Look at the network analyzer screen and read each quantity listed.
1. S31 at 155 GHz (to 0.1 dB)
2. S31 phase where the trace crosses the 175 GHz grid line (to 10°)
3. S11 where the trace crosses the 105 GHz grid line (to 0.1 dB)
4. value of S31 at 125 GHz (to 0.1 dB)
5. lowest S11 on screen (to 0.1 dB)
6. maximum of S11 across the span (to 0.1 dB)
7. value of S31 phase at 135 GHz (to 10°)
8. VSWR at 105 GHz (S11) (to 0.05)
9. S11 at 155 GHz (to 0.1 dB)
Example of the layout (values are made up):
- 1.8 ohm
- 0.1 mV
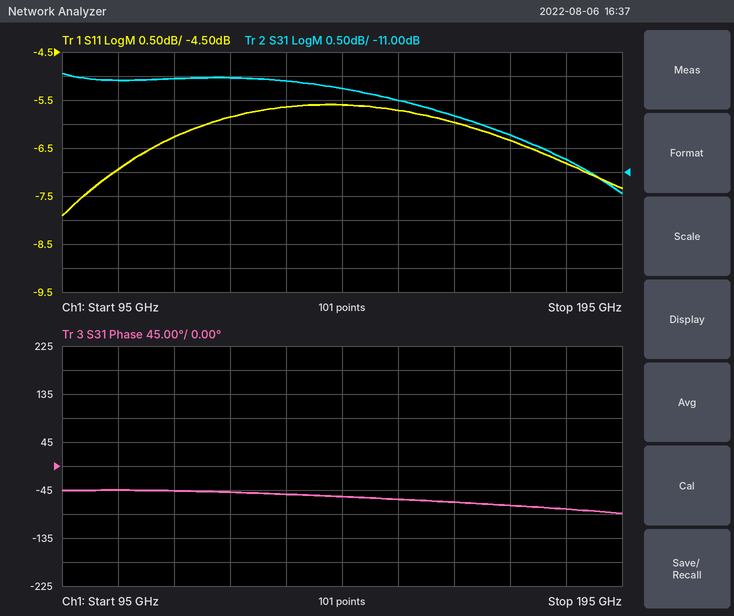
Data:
- -9.5 dB
- -70°
- -6.9 dB
- -9.0 dB
- -7.9 dB
- -5.6 dB
- -50°
- 2.65
- -5.7 dB
